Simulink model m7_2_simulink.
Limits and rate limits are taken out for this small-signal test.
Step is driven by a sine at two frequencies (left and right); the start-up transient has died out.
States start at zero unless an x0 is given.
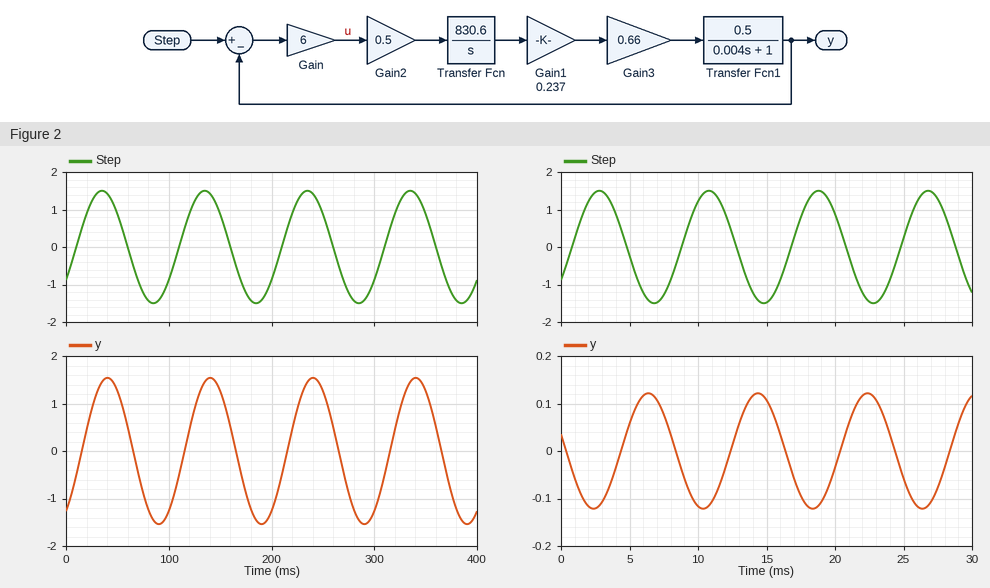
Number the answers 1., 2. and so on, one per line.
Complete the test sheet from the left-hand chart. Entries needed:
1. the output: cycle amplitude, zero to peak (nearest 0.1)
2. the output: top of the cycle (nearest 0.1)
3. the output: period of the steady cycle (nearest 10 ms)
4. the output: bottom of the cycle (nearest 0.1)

1. 1.5
2. 1.5
3. 100 ms
4. -1.5
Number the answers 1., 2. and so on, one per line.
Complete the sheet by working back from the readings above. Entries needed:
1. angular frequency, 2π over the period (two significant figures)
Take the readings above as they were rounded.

1. 0.063 rad/ms
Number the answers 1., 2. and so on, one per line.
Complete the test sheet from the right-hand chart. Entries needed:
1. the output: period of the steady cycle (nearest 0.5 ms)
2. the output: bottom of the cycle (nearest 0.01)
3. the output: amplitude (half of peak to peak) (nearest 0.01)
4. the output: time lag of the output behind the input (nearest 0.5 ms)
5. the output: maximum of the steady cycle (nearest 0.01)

1. 8.0 ms
2. -0.12
3. 0.12
4. 3.5 ms
5. 0.12
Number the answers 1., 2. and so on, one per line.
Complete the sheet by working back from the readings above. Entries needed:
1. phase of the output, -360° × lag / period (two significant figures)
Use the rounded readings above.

1. -160°
